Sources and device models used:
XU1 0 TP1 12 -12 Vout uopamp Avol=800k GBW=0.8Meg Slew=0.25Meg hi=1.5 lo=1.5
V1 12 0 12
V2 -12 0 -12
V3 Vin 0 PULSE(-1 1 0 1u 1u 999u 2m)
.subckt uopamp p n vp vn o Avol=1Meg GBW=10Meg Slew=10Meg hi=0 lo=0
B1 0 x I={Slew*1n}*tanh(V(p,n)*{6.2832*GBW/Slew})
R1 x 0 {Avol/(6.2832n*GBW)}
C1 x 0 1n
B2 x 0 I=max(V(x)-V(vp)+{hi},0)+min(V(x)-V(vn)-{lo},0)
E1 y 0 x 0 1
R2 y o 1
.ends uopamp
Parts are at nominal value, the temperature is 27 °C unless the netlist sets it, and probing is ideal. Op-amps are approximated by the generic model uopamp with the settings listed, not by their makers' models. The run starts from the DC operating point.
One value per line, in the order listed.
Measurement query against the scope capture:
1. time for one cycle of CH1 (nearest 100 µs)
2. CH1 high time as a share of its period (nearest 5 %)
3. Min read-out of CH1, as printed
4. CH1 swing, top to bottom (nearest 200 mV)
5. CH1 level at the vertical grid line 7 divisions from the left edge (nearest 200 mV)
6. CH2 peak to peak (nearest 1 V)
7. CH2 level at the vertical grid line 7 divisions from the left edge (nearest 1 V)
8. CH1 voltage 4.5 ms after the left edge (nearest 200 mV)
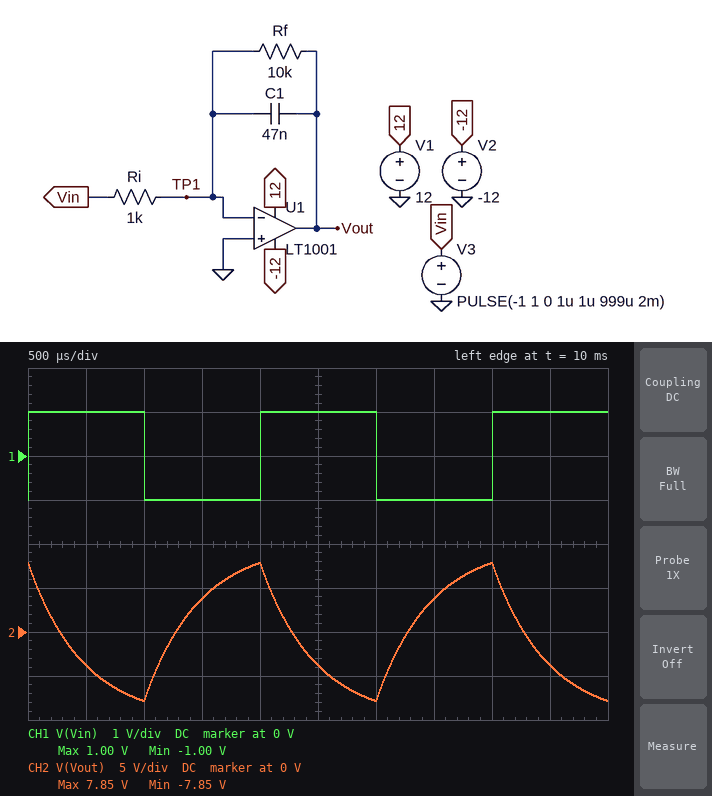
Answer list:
2.0 ms
50 %
-1.00 V
2.0 V
-1.0 V
16 V
4 V
1.0 V
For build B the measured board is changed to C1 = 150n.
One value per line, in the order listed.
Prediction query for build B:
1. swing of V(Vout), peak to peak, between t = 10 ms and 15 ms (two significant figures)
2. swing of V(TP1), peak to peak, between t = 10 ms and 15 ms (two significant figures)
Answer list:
6.4 V
3.5 mV
